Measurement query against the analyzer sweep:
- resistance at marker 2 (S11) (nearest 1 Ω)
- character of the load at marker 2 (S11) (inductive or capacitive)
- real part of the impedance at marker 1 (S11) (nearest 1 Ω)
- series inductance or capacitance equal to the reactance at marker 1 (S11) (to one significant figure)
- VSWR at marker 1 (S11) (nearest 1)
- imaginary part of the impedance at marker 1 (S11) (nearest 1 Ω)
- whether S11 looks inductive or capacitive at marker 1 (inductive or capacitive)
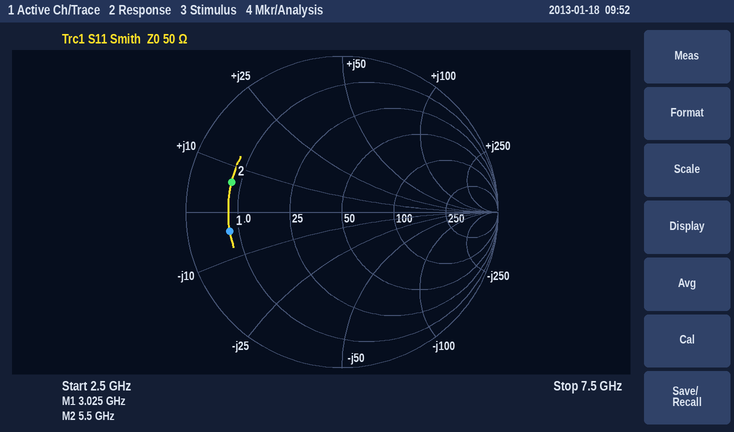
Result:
8 Ω
inductive
8 Ω
10 pF
6
-4 Ω
capacitive
